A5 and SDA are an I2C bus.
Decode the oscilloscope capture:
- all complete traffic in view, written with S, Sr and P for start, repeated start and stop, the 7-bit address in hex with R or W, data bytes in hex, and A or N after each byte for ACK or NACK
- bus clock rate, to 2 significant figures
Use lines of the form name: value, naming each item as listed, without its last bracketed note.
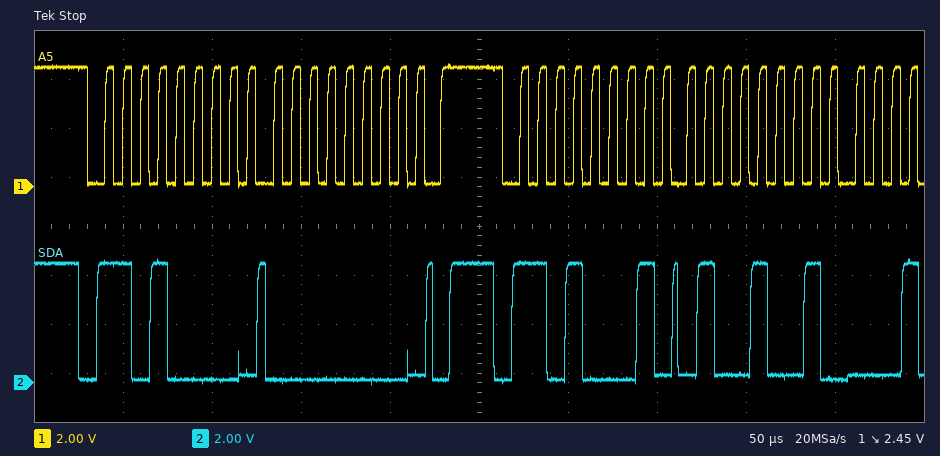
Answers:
all complete traffic in view, written with S, Sr and P for start, repeated start and stop, the 7-bit address in hex with R or W, data bytes in hex, and A or N after each byte for ACK or NACK: S 68W A 00 A P S 68R A 49 A
bus clock rate, to 2 significant figures: 100 kHz
